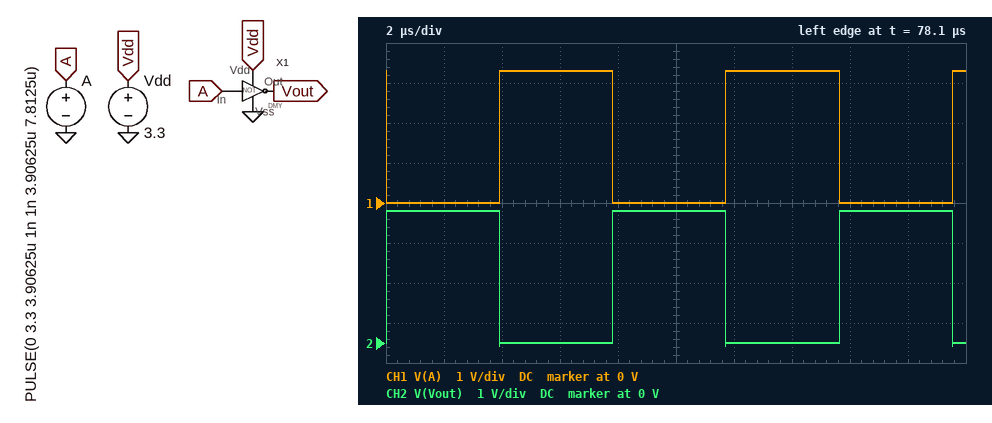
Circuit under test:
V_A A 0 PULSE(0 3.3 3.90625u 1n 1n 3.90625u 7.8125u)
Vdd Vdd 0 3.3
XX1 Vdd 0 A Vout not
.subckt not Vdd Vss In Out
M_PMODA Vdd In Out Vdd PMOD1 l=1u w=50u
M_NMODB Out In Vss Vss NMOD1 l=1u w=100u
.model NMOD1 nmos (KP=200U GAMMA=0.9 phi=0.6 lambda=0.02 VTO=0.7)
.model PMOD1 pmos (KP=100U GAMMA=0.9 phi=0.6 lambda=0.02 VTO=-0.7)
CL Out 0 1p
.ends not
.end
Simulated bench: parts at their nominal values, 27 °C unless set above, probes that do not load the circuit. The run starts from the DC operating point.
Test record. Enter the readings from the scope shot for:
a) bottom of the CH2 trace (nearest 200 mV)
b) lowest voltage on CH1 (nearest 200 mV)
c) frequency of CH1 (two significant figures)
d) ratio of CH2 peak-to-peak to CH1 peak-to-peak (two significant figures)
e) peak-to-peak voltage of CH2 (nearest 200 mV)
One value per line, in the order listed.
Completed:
0 V
0 V
130 kHz
1.0
3.4 V
